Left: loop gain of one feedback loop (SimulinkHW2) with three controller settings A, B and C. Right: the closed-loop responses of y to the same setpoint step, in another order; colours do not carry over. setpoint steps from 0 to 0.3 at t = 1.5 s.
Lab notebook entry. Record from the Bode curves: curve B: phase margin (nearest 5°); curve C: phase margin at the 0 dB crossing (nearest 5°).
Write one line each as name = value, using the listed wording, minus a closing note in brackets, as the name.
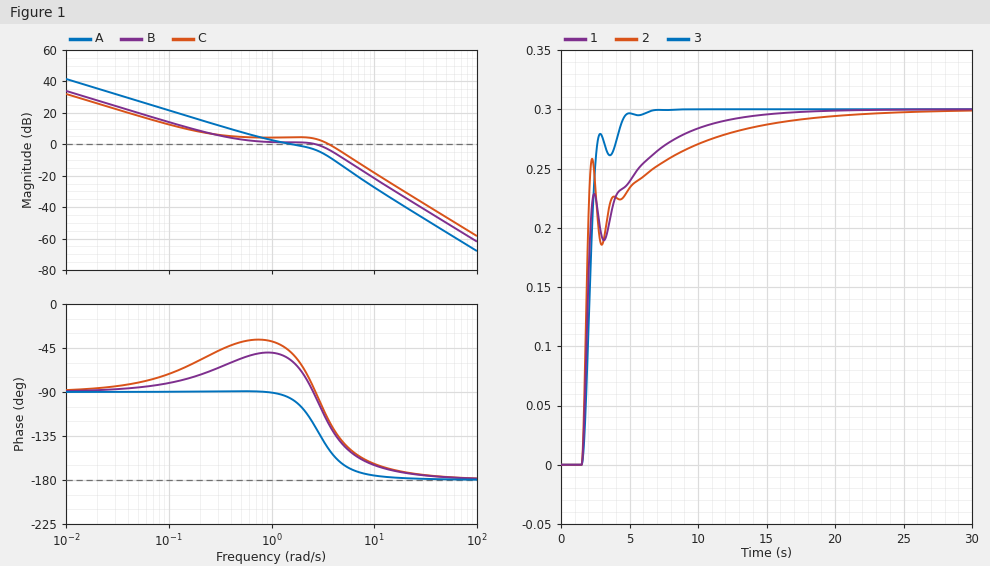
curve B: phase margin = 85°
curve C: phase margin at the 0 dB crossing = 60°
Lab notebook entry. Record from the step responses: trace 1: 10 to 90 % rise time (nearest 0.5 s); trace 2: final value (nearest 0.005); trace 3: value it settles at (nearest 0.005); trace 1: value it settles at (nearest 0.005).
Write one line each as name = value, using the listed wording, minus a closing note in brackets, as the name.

trace 1: 10 to 90 % rise time = 6.0 s
trace 2: final value = 0.300
trace 3: value it settles at = 0.300
trace 1: value it settles at = 0.300
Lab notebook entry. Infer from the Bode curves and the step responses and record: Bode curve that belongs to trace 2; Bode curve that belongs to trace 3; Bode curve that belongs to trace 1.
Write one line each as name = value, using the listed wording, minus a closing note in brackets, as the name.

Bode curve that belongs to trace 2 = C
Bode curve that belongs to trace 3 = A
Bode curve that belongs to trace 1 = B
